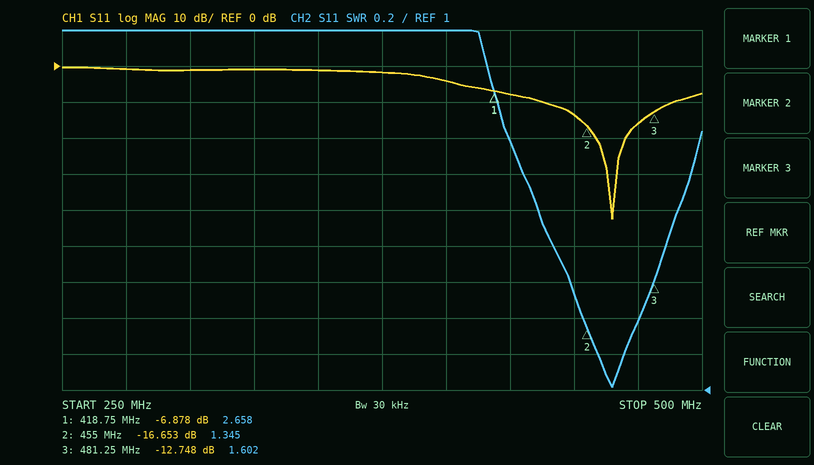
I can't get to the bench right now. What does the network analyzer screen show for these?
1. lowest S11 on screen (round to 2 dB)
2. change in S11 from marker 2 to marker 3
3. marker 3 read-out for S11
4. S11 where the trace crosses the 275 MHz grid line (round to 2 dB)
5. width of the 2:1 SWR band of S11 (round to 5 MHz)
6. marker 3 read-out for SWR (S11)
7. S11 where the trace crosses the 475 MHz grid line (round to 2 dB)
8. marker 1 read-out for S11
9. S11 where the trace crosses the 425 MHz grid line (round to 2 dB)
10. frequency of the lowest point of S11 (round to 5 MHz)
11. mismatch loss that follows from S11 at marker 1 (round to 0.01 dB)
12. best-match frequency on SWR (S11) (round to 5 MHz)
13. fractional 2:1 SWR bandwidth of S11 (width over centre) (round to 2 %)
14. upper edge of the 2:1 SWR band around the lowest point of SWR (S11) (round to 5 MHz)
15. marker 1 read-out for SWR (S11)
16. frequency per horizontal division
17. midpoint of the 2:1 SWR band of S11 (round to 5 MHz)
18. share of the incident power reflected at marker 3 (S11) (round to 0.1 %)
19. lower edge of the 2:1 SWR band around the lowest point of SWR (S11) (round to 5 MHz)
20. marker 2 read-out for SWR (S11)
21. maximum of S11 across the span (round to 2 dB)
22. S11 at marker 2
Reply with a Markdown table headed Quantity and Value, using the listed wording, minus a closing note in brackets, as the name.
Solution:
| Quantity | Value |
|---|---|
| lowest S11 on screen | -42 dB |
| change in S11 from marker 2 to marker 3 | 3.905 dB |
| marker 3 read-out for S11 | -12.748 dB |
| S11 where the trace crosses the 275 MHz grid line | 0 dB |
| width of the 2:1 SWR band of S11 | 55 MHz |
| marker 3 read-out for SWR | 1.602 |
| S11 where the trace crosses the 475 MHz grid line | -16 dB |
| marker 1 read-out for S11 | -6.878 dB |
| S11 where the trace crosses the 425 MHz grid line | -8 dB |
| frequency of the lowest point of S11 | 465 MHz |
| mismatch loss that follows from S11 at marker 1 | 1.00 dB |
| best-match frequency on SWR (S11) | 465 MHz |
| fractional 2:1 SWR bandwidth of S11 (width over centre) | 12 % |
| upper edge of the 2:1 SWR band around the lowest point of SWR (S11) | 490 MHz |
| marker 1 read-out for SWR | 2.658 |
| frequency per horizontal division | 25 MHz |
| midpoint of the 2:1 SWR band of S11 | 465 MHz |
| share of the incident power reflected at marker 3 (S11) | 5.3 % |
| lower edge of the 2:1 SWR band around the lowest point of SWR (S11) | 435 MHz |
| marker 2 read-out for SWR | 1.345 |
| maximum of S11 across the span | 0 dB |
| S11 at marker 2 | -16.653 dB |
